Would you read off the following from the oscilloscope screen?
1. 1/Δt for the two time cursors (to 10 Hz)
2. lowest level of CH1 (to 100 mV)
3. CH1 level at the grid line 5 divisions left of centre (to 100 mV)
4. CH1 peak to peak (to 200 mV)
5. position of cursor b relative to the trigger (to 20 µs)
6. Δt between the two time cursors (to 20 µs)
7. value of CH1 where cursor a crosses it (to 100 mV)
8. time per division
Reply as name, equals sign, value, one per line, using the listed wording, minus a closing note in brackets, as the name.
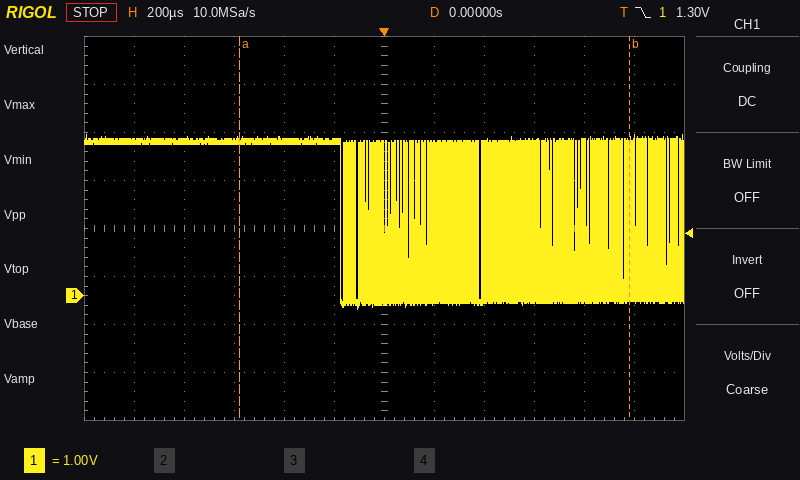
1/Δt for the two time cursors = 640 Hz
lowest level of CH1 = -300 mV
CH1 level at the grid line 5 divisions left of centre = 3.2 V
CH1 peak to peak = 3.6 V
position of cursor b relative to the trigger = +980 µs
Δt between the two time cursors = 1.56 ms
value of CH1 where cursor a crosses it = 3.2 V
time per division = 200 µs
